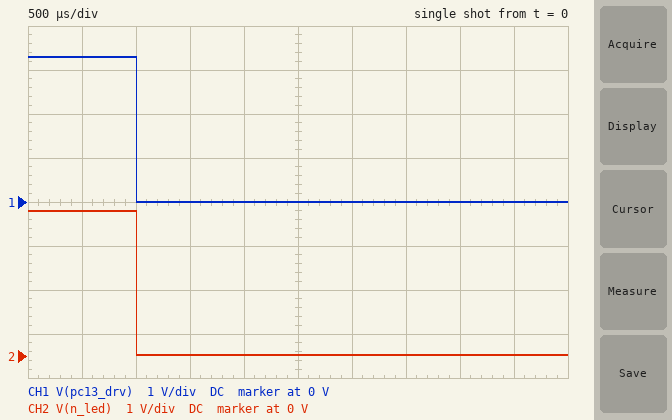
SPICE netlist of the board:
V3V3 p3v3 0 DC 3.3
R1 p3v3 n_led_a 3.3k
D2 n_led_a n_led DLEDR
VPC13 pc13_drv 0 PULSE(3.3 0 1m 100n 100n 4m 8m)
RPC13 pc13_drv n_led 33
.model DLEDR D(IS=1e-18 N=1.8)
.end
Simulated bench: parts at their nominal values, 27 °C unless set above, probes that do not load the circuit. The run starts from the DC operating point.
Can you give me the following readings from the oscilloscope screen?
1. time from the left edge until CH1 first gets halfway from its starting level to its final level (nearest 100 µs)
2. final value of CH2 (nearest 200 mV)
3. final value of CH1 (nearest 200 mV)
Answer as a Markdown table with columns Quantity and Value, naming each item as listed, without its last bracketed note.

| Quantity | Value |
|---|---|
| time from the left edge until CH1 first gets halfway from its starting level to its final level | 1.0 ms |
| final value of CH2 | 0 V |
| final value of CH1 | 0 V |
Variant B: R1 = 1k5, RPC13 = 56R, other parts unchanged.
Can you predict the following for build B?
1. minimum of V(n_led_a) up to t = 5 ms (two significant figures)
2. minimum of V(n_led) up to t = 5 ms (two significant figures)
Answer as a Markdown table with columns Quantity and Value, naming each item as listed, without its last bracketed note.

| Quantity | Value |
|---|---|
| minimum of V(n_led_a) up to t = 5 ms | 1.7 V |
| minimum of V(n_led) up to t = 5 ms | 61 mV |
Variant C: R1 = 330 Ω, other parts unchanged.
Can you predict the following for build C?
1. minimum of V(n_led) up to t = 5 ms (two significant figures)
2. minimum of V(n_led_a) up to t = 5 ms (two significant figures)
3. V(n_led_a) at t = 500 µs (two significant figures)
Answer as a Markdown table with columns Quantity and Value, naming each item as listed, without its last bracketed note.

| Quantity | Value |
|---|---|
| minimum of V(n_led) up to t = 5 ms | 150 mV |
| minimum of V(n_led_a) up to t = 5 ms | 1.8 V |
| V(n_led_a) at t = 500 µs | 3.3 V |
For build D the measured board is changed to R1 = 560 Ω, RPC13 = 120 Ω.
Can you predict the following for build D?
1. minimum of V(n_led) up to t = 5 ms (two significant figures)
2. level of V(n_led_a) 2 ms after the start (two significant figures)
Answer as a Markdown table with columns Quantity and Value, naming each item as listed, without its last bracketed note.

| Quantity | Value |
|---|---|
| minimum of V(n_led) up to t = 5 ms | 290 mV |
| level of V(n_led_a) 2 ms after the start | 1.9 V |
